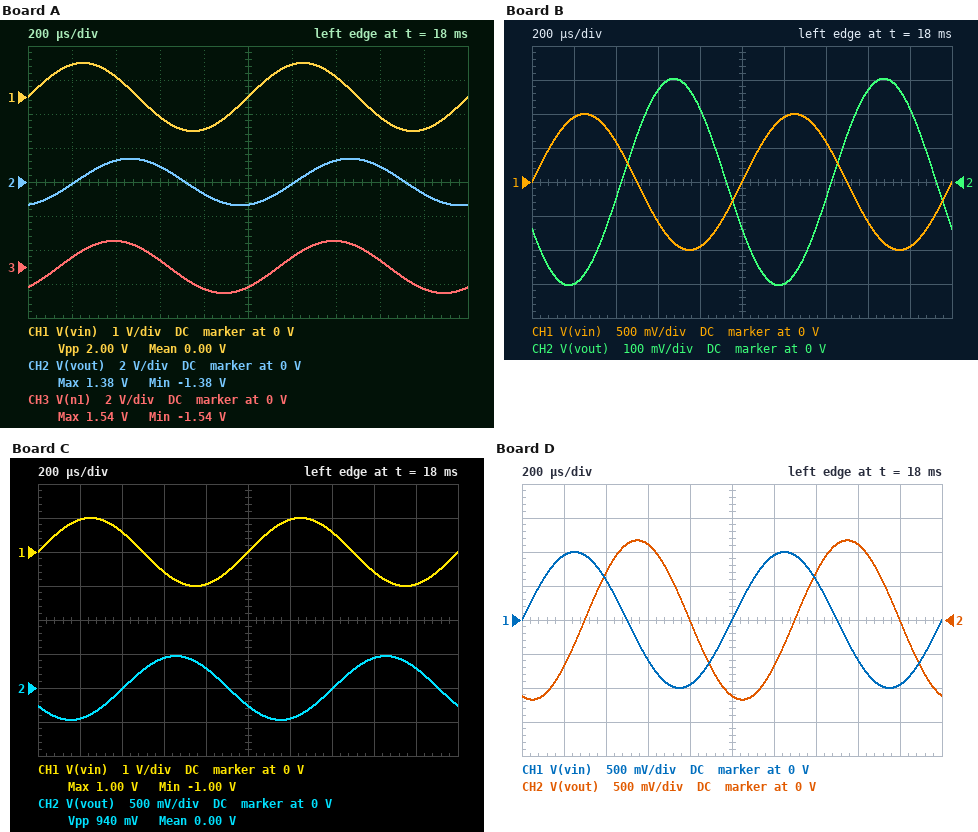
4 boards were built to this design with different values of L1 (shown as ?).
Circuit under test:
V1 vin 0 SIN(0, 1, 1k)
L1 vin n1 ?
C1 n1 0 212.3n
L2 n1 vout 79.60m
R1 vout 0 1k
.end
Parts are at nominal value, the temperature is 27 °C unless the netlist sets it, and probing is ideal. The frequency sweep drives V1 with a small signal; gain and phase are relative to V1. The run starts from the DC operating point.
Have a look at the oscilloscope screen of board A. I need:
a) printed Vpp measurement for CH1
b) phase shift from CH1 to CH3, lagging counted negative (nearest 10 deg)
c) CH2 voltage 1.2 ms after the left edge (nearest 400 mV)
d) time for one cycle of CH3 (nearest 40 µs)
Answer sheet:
2.00 V
-50 deg
0 V
1.00 ms
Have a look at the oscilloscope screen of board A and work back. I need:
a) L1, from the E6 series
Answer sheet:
100 mH
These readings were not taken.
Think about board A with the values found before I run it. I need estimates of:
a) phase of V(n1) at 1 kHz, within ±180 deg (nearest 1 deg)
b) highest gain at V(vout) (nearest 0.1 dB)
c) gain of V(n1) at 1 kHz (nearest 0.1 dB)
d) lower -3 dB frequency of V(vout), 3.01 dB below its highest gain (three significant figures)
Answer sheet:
-51 deg
3.6 dB
3.7 dB
516 Hz
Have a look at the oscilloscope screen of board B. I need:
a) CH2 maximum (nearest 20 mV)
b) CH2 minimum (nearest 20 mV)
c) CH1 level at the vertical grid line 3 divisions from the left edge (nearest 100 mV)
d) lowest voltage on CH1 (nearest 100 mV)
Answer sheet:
300 mV
-300 mV
-600 mV
-1.0 V
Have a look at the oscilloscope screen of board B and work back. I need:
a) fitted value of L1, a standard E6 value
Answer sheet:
470 mH
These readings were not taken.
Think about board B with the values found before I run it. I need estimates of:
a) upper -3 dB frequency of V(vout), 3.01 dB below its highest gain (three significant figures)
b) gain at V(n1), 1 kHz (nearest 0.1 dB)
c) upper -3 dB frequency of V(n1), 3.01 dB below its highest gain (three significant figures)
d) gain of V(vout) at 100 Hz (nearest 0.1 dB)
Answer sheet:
464 Hz
-9.4 dB
487 Hz
-0.2 dB
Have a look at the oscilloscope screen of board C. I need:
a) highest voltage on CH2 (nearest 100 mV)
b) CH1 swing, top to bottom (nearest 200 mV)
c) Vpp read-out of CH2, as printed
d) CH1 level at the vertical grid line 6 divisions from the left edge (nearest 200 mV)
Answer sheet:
500 mV
2.0 V
940 mV
1.0 V
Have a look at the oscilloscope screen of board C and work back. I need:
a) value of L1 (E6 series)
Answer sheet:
330 mH
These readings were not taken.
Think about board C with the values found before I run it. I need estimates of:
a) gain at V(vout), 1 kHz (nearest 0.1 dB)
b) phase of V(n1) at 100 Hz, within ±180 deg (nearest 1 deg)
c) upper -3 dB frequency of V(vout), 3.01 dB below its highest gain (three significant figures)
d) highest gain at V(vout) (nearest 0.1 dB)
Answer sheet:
-6.6 dB
-12 deg
725 Hz
0 dB
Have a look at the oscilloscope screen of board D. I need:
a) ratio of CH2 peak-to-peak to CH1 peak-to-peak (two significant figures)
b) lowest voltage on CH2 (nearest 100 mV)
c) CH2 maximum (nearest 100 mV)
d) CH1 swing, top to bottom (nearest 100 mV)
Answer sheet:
1.2
-1.2 V
1.2 V
2.0 V
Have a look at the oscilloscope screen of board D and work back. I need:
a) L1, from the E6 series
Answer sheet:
150 mH
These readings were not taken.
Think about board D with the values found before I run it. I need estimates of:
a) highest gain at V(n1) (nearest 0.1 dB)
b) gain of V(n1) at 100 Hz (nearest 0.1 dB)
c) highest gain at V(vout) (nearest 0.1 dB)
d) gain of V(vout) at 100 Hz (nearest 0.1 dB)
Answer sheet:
2.4 dB
0 dB
1.5 dB
0 dB
